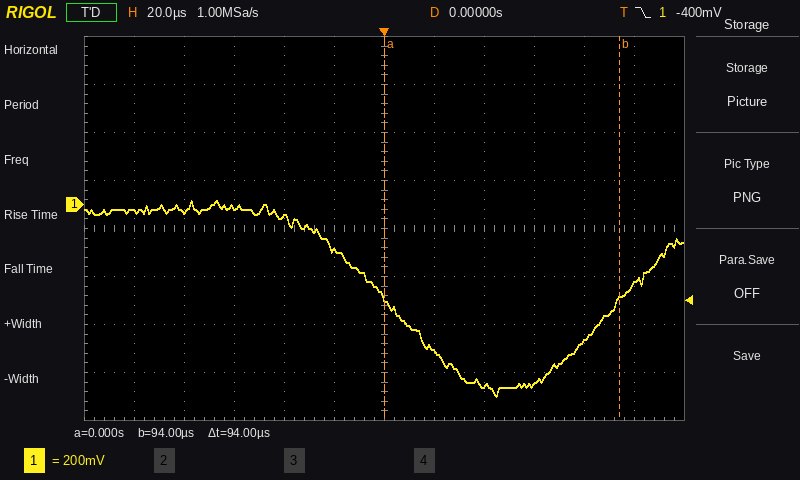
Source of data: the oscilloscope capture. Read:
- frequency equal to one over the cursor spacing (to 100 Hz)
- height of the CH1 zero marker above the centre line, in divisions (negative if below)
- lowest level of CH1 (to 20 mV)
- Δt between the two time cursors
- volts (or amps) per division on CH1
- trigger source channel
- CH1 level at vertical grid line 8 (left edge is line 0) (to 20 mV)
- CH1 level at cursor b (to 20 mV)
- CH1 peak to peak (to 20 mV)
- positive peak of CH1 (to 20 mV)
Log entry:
10.6 kHz
+0.5 div
-800 mV
94 µs
200 mV
CH1
-760 mV
-400 mV
820 mV
20 mV
